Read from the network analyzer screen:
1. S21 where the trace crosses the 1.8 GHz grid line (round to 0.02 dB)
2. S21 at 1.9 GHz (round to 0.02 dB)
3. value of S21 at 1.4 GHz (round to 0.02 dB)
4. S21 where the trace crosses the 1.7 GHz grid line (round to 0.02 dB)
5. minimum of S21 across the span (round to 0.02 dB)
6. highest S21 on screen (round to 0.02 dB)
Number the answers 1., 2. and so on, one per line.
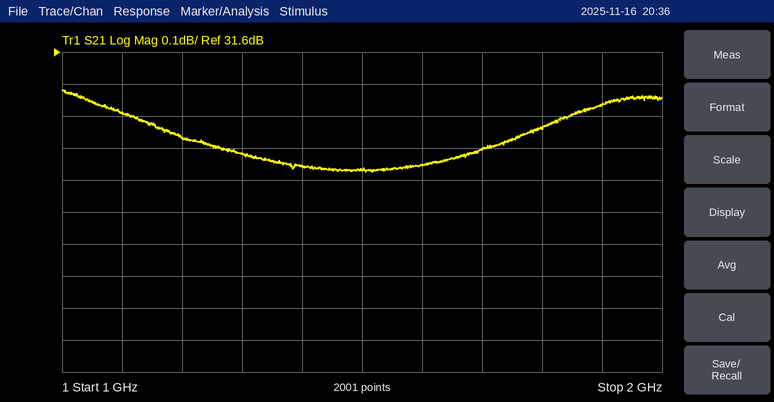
1. 31.36 dB
2. 31.44 dB
3. 31.24 dB
4. 31.30 dB
5. 31.22 dB
6. 31.48 dB
